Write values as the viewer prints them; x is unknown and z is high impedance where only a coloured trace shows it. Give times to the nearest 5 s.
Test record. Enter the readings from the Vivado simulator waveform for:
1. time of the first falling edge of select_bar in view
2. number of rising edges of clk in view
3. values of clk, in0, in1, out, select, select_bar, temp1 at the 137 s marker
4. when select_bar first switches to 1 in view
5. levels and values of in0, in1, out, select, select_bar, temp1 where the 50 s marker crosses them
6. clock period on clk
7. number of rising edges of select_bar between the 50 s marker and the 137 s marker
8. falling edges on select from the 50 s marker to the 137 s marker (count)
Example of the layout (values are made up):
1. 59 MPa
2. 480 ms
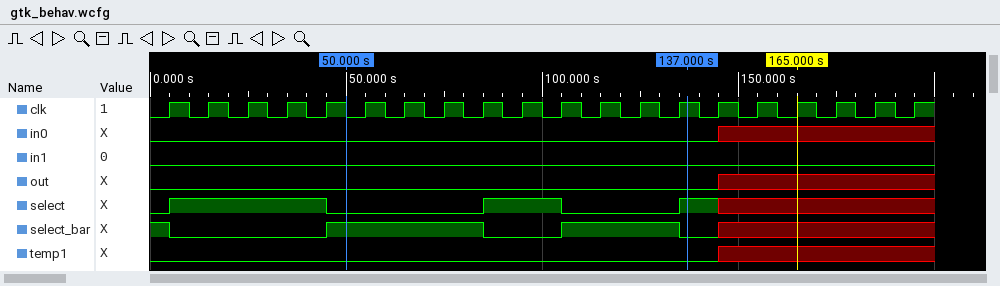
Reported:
1. 5 s
2. 20
3. clk=1, in0=0, in1=0, out=0, select=1, select_bar=0, temp1=0
4. 45 s
5. in0=0, in1=0, out=0, select=0, select_bar=1, temp1=0
6. 10 s
7. 1
8. 1
